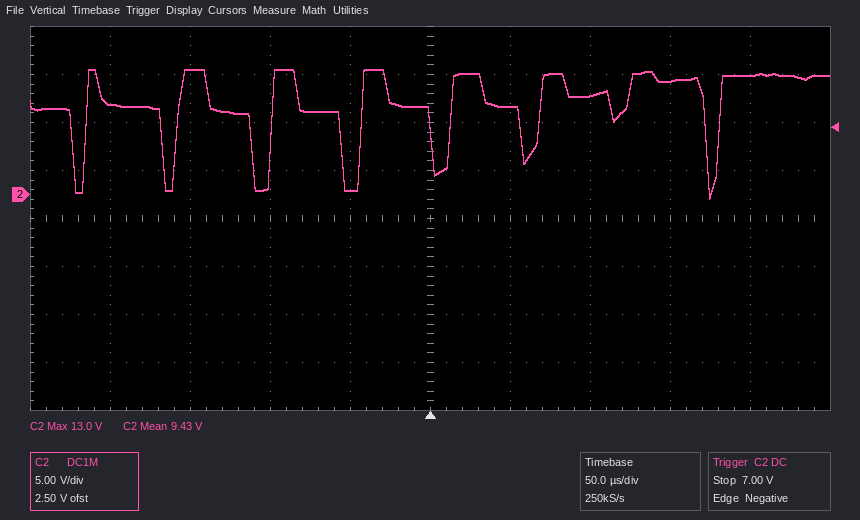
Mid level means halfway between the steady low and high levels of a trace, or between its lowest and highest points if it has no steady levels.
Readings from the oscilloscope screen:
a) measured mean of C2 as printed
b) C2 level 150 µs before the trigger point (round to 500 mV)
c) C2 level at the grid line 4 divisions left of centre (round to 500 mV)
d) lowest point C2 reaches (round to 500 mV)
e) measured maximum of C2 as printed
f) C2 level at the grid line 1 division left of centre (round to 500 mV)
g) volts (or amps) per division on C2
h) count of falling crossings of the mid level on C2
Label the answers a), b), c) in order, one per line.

a) 9.43 V
b) 13.0 V
c) 9.5 V
d) -500 mV
e) 13.0 V
f) 500 mV
g) 5 V
h) 7
